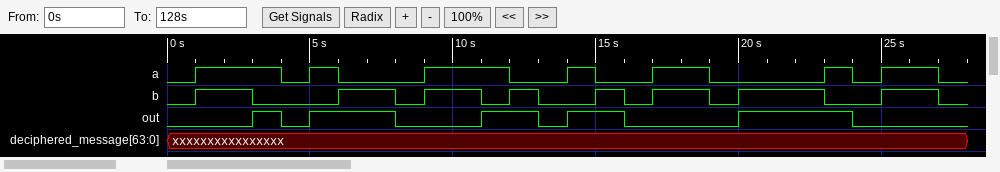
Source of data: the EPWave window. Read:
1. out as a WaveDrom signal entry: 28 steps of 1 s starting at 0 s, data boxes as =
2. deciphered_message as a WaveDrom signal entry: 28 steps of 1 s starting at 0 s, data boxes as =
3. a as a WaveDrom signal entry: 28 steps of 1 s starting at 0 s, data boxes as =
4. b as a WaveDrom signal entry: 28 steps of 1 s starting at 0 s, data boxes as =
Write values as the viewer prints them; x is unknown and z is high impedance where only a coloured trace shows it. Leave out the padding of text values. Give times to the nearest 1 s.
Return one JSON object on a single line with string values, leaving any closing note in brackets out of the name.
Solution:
{"out as a WaveDrom signal entry: 28 steps of 1 s starting at 0 s, data boxes as =": "{name: 'out', wave: '0..101..0..1.01.0...1...0...'}", "deciphered_message as a WaveDrom signal entry: 28 steps of 1 s starting at 0 s, data boxes as =": "{name: 'deciphered_message', wave: 'x...........................'}", "a as a WaveDrom signal entry: 28 steps of 1 s starting at 0 s, data boxes as =": "{name: 'a', wave: '01..010..1..0.10.1.0...101.0'}", "b as a WaveDrom signal entry: 28 steps of 1 s starting at 0 s, data boxes as =": "{name: 'b', wave: '01.0..1.01.010.101.01..0.1.0'}"}
